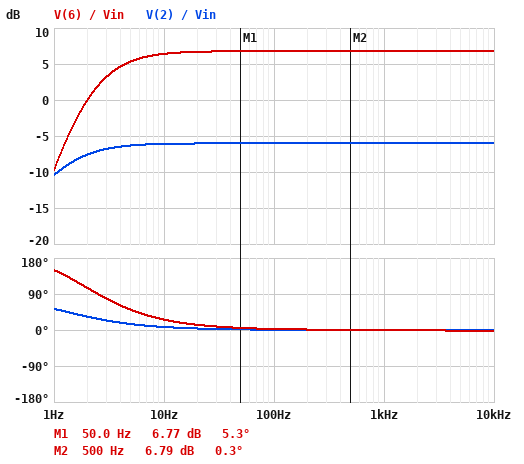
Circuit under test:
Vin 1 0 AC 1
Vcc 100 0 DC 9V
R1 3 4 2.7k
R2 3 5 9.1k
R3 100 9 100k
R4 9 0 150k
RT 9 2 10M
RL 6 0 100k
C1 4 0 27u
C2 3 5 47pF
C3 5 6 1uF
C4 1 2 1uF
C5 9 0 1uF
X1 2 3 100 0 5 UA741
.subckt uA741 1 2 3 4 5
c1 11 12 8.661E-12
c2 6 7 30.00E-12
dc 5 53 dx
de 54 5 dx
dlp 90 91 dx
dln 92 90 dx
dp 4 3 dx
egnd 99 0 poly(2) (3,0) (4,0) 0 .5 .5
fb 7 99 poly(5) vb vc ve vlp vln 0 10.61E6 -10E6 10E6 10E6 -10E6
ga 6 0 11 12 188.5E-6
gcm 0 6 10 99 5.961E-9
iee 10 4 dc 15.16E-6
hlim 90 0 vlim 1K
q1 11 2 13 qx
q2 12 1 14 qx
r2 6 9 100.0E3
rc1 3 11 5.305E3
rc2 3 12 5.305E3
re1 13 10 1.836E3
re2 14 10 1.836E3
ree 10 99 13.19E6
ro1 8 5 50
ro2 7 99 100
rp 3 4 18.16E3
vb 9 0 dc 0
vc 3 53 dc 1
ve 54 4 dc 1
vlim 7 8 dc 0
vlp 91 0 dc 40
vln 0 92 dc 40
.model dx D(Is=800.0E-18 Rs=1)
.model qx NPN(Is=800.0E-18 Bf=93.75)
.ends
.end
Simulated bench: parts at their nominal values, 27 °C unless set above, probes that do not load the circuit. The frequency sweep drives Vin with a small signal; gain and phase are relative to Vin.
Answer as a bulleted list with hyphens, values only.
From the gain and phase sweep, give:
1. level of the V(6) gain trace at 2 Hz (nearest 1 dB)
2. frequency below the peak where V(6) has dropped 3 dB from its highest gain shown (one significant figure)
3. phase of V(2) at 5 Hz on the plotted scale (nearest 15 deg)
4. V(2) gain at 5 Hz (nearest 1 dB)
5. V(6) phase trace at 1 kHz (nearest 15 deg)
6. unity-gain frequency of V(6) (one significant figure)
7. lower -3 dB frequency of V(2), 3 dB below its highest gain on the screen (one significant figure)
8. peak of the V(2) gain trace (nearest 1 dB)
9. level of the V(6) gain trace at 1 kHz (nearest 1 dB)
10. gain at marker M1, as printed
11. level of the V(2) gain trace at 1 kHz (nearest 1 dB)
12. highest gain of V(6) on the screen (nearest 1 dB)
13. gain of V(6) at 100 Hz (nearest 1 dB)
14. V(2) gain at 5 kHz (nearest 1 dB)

- 0 dB
- 3 Hz
- 15 deg
- -6 dB
- 0 deg
- 2 Hz
- 1 Hz
- -6 dB
- 7 dB
- 6.77 dB
- -6 dB
- 7 dB
- 7 dB
- -6 dB
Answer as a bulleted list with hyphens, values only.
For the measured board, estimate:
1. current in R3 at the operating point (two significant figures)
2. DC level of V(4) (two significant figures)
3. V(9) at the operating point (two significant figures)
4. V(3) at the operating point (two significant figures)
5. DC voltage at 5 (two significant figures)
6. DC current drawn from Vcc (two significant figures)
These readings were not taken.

- 36 µA
- 5.4 V
- 5.4 V
- 5.4 V
- 5.4 V
- 550 µA
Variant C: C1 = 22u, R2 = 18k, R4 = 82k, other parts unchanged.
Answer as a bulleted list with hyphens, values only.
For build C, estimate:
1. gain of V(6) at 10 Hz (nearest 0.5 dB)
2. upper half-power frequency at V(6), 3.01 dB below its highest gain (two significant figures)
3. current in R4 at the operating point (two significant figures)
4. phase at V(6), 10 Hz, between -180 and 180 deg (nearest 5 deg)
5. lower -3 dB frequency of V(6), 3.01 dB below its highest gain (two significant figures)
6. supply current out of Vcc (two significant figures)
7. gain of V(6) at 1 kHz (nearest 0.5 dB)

- 11.0 dB
- 82 kHz
- 49 µA
- 30 deg
- 4.0 Hz
- 560 µA
- 11.5 dB
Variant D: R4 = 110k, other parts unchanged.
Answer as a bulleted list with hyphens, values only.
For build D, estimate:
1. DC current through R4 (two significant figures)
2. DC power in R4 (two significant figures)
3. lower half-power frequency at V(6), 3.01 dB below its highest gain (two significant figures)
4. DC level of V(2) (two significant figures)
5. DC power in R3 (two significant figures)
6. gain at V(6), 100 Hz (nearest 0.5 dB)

- 43 µA
- 200 µW
- 3.4 Hz
- 4.7 V
- 180 µW
- 7.0 dB
